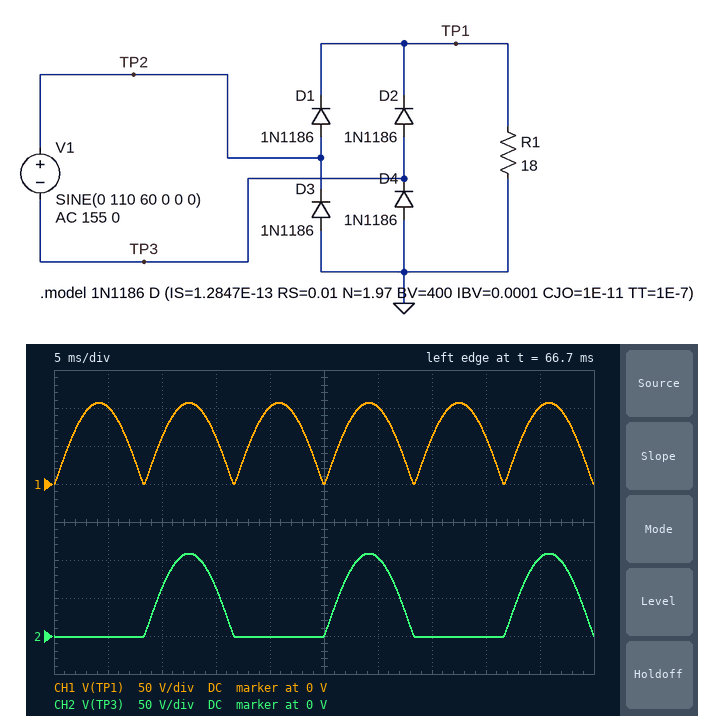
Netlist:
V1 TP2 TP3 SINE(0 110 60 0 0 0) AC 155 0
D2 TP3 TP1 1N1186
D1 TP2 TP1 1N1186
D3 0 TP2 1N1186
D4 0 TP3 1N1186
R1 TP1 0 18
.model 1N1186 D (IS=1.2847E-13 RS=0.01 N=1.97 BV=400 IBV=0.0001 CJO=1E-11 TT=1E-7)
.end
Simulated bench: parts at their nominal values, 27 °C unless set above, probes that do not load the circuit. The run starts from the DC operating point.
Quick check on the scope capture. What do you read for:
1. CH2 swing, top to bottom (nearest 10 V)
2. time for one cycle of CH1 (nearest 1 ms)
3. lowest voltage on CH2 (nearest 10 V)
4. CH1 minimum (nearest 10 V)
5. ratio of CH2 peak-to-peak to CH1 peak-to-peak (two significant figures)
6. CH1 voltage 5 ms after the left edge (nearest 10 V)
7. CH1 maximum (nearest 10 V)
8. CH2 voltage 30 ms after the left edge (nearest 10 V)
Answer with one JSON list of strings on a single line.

["110 V", "8 ms", "0 V", "0 V", "1.0", "100 V", "110 V", "100 V"]
